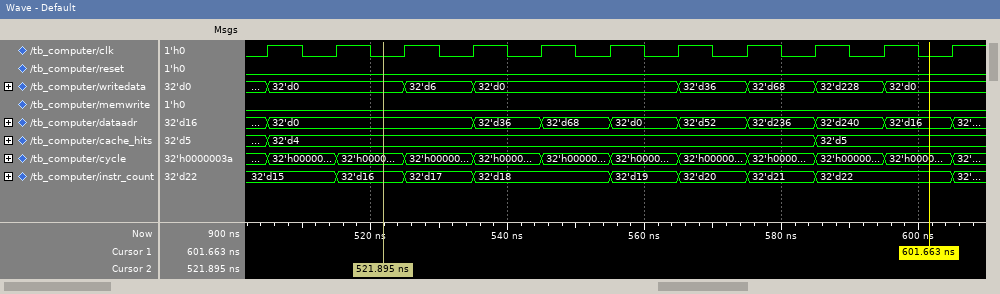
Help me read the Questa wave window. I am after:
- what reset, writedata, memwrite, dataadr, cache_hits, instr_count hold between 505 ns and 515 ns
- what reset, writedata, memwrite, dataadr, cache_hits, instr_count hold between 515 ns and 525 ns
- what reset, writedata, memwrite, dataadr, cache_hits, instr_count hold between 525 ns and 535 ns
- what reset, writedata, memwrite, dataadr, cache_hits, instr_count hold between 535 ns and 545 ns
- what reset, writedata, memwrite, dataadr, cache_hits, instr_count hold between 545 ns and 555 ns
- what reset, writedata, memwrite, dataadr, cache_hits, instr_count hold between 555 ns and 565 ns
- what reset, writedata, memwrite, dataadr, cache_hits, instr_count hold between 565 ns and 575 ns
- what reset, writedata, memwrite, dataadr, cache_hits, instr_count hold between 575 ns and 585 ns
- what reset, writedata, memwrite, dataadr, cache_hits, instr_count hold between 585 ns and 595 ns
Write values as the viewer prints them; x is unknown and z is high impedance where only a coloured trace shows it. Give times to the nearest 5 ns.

reset=0, writedata=32'd0, memwrite=0, dataadr=32'd0, cache_hits=32'd4, instr_count=32'd15
reset=0, writedata=32'd0, memwrite=0, dataadr=32'd0, cache_hits=32'd4, instr_count=32'd16
reset=0, writedata=32'd6, memwrite=0, dataadr=32'd0, cache_hits=32'd4, instr_count=32'd17
reset=0, writedata=32'd0, memwrite=0, dataadr=32'd36, cache_hits=32'd4, instr_count=32'd18
reset=0, writedata=32'd0, memwrite=0, dataadr=32'd68, cache_hits=32'd4, instr_count=32'd18
reset=0, writedata=32'd0, memwrite=0, dataadr=32'd0, cache_hits=32'd4, instr_count=32'd19
reset=0, writedata=32'd36, memwrite=0, dataadr=32'd52, cache_hits=32'd4, instr_count=32'd20
reset=0, writedata=32'd68, memwrite=0, dataadr=32'd236, cache_hits=32'd4, instr_count=32'd21
reset=0, writedata=32'd228, memwrite=0, dataadr=32'd240, cache_hits=32'd5, instr_count=32'd22
